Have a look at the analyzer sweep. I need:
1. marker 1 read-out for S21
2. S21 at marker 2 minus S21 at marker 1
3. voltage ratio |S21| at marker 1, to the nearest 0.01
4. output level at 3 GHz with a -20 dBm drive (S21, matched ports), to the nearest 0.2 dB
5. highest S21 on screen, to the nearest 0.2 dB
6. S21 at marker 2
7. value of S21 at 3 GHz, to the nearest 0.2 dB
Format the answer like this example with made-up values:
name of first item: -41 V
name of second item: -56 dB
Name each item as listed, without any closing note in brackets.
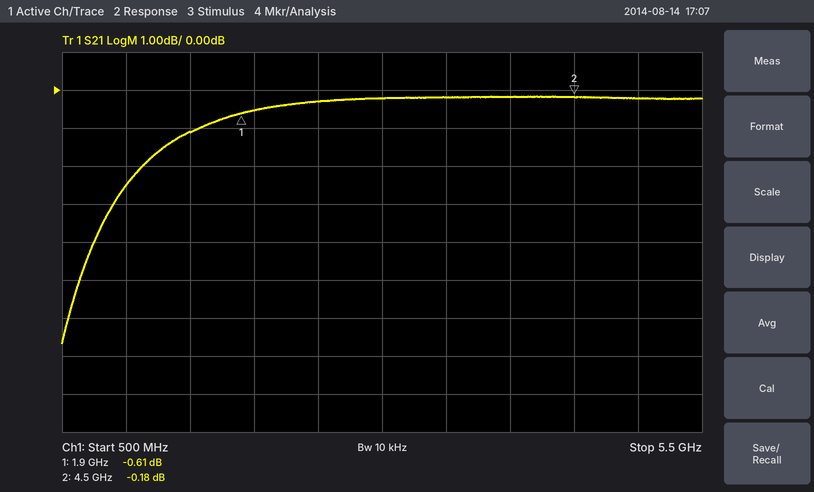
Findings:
marker 1 read-out for S21: -0.61 dB
S21 at marker 2 minus S21 at marker 1: 0.43 dB
voltage ratio |S21| at marker 1, to the nearest 0.01: 0.93
output level at 3 GHz with a -20 dBm drive (S21, matched ports), to the nearest 0.2 dB: -20.2 dBm
highest S21 on screen, to the nearest 0.2 dB: -0.2 dB
S21 at marker 2: -0.18 dB
value of S21 at 3 GHz, to the nearest 0.2 dB: -0.2 dB
